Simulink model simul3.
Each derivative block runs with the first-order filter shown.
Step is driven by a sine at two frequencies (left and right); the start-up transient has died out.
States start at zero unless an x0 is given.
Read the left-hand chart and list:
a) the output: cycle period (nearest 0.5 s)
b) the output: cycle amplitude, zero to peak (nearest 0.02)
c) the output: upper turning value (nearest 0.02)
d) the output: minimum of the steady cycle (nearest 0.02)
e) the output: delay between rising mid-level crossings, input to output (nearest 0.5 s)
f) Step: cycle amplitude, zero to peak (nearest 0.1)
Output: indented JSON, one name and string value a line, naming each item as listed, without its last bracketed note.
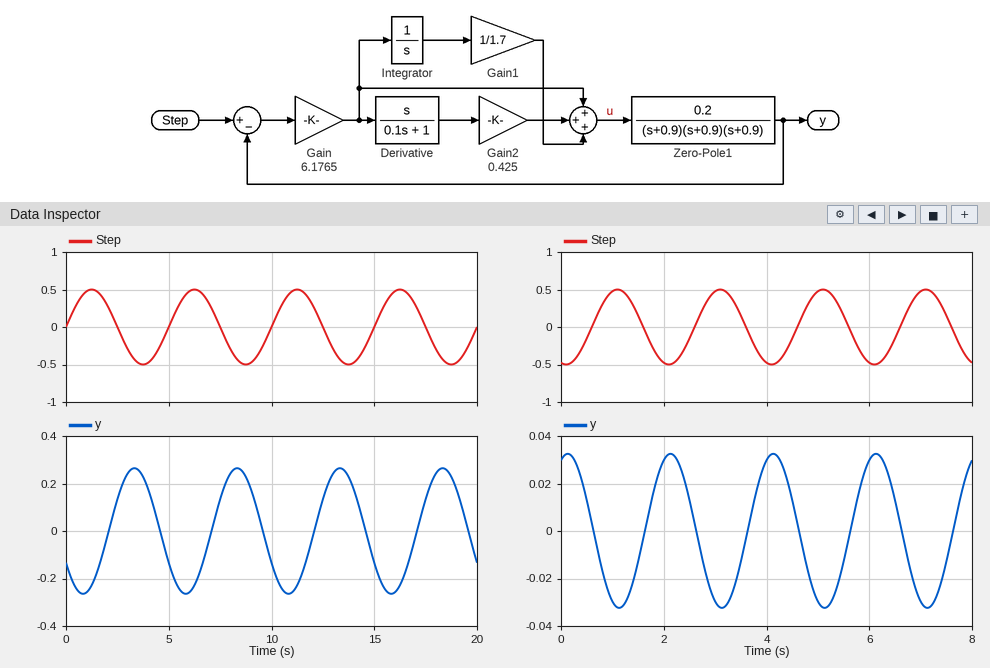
{
  "the output: cycle period": "5.0 s",
  "the output: cycle amplitude, zero to peak": "0.26",
  "the output: upper turning value": "0.26",
  "the output: minimum of the steady cycle": "-0.26",
  "the output: delay between rising mid-level crossings, input to output": "2.0 s",
  "Step: cycle amplitude, zero to peak": "0.5"
}
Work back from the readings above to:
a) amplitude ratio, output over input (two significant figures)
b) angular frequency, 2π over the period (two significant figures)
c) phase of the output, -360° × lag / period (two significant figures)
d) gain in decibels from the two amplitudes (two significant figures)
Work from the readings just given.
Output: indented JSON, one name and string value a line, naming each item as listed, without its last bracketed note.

{
  "amplitude ratio, output over input": "0.52",
  "angular frequency, 2π over the period": "1.3 rad/s",
  "phase of the output, -360° × lag / period": "-140°",
  "gain in decibels from the two amplitudes": "-5.7 dB"
}
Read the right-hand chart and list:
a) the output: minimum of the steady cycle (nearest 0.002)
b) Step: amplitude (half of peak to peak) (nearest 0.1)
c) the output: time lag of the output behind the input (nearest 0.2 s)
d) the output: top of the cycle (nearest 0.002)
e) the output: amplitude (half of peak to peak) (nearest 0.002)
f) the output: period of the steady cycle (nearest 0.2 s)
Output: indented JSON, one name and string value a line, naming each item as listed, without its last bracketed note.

{
  "the output: minimum of the steady cycle": "-0.032",
  "Step: amplitude (half of peak to peak)": "0.5",
  "the output: time lag of the output behind the input": "1.0 s",
  "the output: top of the cycle": "0.032",
  "the output: amplitude (half of peak to peak)": "0.032",
  "the output: period of the steady cycle": "2.0 s"
}
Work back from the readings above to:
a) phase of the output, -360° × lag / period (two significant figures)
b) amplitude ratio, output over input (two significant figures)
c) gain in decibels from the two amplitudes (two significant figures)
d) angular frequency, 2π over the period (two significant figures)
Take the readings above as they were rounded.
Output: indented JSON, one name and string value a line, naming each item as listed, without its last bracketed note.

{
  "phase of the output, -360° × lag / period": "-180°",
  "amplitude ratio, output over input": "0.064",
  "gain in decibels from the two amplitudes": "-24 dB",
  "angular frequency, 2π over the period": "3.1 rad/s"
}
